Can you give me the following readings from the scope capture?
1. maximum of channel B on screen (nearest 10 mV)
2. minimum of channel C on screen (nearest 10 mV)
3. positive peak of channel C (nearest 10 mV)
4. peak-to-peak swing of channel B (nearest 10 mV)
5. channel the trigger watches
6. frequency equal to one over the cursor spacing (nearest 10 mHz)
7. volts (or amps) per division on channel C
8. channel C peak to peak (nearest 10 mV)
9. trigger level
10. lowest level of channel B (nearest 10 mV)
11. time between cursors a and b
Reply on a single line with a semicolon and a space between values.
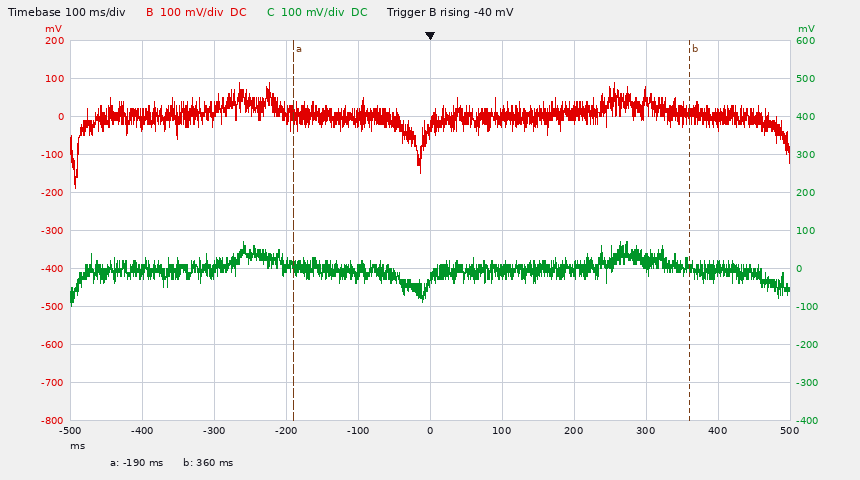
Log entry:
90 mV; -100 mV; 70 mV; 280 mV; channel B; 1.82 Hz; 100 mV; 170 mV; -40 mV; -190 mV; 550 ms
